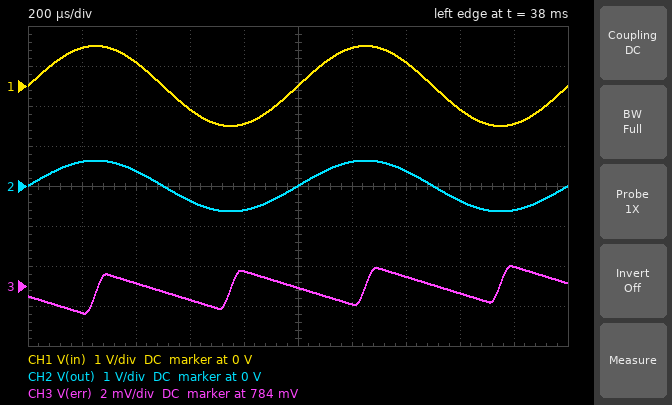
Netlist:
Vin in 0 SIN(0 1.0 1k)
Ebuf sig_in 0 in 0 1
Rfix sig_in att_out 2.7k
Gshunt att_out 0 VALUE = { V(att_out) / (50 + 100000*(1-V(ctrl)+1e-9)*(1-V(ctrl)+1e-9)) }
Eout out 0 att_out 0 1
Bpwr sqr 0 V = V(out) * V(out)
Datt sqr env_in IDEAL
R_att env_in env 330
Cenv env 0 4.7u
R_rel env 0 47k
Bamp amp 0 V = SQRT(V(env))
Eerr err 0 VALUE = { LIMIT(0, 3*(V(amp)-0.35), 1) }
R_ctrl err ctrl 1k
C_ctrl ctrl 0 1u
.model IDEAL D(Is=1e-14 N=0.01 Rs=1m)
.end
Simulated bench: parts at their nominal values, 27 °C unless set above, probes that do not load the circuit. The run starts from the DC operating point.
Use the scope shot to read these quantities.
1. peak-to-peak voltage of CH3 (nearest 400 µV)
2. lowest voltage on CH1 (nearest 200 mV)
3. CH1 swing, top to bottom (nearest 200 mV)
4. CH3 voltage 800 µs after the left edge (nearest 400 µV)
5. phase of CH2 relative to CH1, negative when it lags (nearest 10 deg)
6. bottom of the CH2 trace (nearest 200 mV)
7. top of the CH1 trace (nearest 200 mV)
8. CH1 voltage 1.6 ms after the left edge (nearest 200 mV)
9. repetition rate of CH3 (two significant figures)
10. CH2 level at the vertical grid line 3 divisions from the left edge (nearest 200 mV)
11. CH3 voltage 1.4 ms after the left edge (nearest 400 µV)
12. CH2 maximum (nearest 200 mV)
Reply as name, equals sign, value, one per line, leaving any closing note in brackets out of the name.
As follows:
peak-to-peak voltage of CH3 = 2.4 mV
lowest voltage on CH1 = -1.0 V
CH1 swing, top to bottom = 2.0 V
CH3 voltage 800 µs after the left edge = 784.8 mV
phase of CH2 relative to CH1, negative when it lags = 0 deg
bottom of the CH2 trace = -600 mV
top of the CH1 trace = 1.0 V
CH1 voltage 1.6 ms after the left edge = -600 mV
repetition rate of CH3 = 2.0 kHz
CH2 level at the vertical grid line 3 divisions from the left edge = -400 mV
CH3 voltage 1.4 ms after the left edge = 784.4 mV
CH2 maximum = 600 mV
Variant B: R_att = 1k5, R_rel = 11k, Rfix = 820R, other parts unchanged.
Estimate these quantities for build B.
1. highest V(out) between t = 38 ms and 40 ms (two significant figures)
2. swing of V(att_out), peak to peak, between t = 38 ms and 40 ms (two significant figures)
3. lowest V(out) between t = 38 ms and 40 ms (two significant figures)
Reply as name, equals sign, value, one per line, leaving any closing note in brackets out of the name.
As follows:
highest V(out) between t = 38 ms and 40 ms = 780 mV
swing of V(att_out), peak to peak, between t = 38 ms and 40 ms = 1.6 V
lowest V(out) between t = 38 ms and 40 ms = -780 mV
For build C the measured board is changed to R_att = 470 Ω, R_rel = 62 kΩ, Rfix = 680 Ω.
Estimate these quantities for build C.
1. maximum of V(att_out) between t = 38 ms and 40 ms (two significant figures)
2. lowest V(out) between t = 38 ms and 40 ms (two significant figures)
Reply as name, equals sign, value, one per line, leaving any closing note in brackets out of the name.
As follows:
maximum of V(att_out) between t = 38 ms and 40 ms = 670 mV
lowest V(out) between t = 38 ms and 40 ms = -670 mV
